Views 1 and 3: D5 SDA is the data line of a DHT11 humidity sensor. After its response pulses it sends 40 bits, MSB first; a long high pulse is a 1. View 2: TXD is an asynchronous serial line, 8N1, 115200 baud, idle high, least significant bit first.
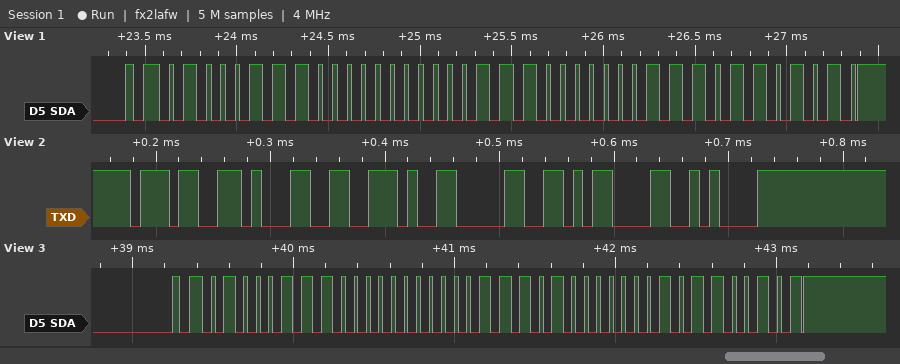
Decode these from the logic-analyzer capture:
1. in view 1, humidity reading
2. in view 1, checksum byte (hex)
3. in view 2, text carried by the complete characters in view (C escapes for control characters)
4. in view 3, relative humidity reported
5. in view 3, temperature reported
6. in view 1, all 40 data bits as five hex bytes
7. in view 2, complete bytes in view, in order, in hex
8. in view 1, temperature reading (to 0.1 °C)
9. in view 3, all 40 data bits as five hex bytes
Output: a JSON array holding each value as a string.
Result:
["71 %", "0x6A", "\"71.0\\r\\n\"", "71 %", "29.1 °C", "47 00 1C 07 6A", "37 31 2E 30 0D 0A", "28.7 °C", "47 00 1D 01 65"]
